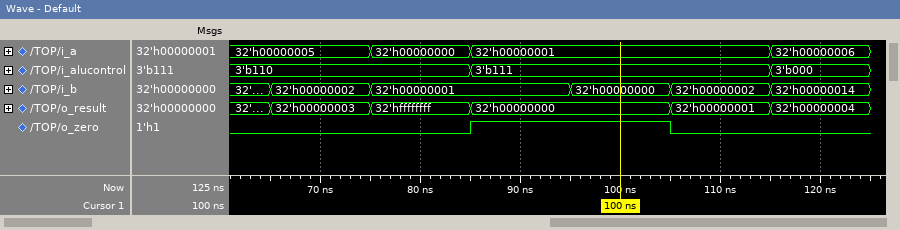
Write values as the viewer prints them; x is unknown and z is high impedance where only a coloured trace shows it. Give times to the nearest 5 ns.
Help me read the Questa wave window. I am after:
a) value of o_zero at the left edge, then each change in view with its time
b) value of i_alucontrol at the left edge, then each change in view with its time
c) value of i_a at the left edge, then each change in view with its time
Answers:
0, 1 at 85 ns, 0 at 105 ns
3'b110, 3'b111 at 85 ns, 3'b000 at 115 ns
32'h00000005, 32'h00000000 at 75 ns, 32'h00000001 at 85 ns, 32'h00000006 at 115 ns
